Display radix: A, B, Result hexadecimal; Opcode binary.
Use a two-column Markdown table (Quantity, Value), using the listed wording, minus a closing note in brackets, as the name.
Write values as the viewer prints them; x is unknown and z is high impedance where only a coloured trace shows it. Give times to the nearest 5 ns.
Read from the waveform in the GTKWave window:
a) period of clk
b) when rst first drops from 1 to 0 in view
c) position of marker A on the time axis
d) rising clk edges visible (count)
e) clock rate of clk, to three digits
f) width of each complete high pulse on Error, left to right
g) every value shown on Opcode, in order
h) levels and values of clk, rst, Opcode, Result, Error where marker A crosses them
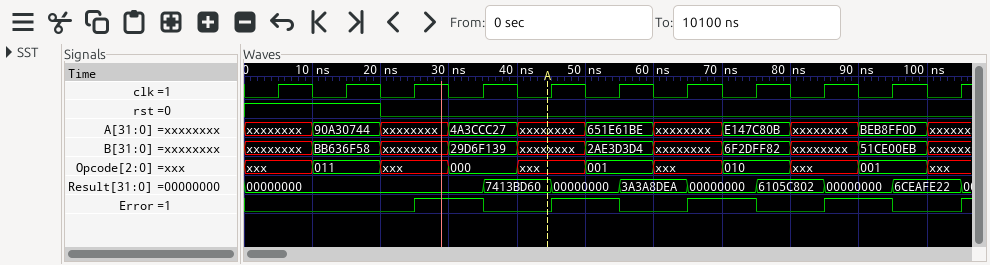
| Quantity | Value |
|---|---|
| period of clk | 10 ns |
| when rst first drops from 1 to 0 in view | 20 ns |
| position of marker A on the time axis | 45 ns |
| rising clk edges visible | 11 |
| clock rate of clk, to three digits | 100 MHz |
| width of each complete high pulse on Error, left to right | 10 ns, 10 ns, 10 ns, 10 ns |
| every value shown on Opcode, in order | xxx, 011, xxx, 000, xxx, 001, xxx, 010, xxx, 001, xxx |
| levels and values of clk, rst, Opcode, Result, Error where marker A crosses them | clk=0, rst=0, Opcode=xxx, Result=7413BD60, Error=0 |
